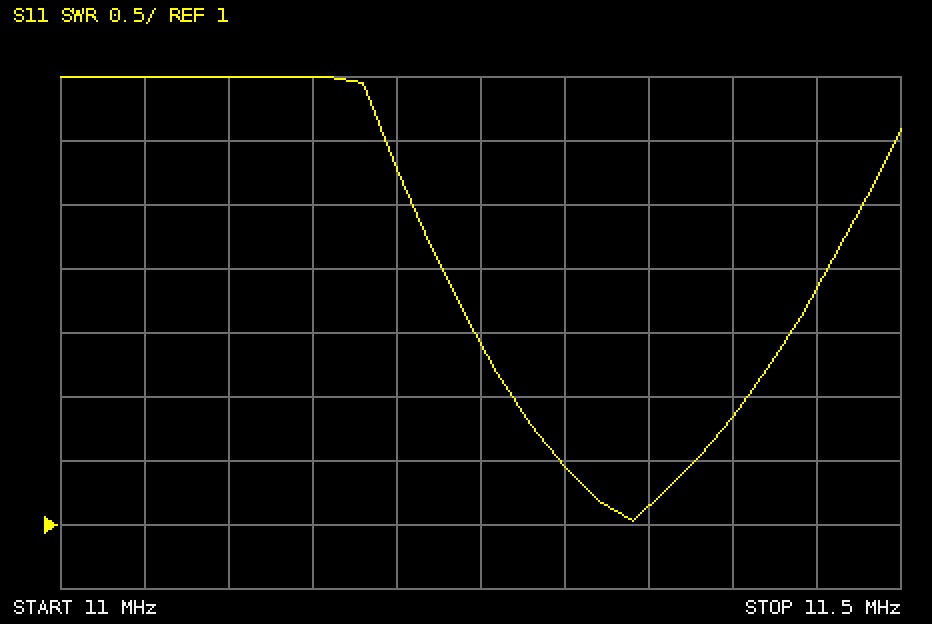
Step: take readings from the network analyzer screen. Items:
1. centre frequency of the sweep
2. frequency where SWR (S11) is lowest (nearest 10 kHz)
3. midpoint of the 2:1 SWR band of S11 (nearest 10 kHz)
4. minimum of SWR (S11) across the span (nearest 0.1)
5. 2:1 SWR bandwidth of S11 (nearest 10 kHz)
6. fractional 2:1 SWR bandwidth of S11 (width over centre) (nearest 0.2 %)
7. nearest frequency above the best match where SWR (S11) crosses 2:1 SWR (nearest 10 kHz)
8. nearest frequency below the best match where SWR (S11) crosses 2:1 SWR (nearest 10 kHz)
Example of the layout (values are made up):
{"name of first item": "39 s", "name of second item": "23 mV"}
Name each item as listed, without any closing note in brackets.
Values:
{"centre frequency of the sweep": "11.25 MHz", "frequency where SWR (S11) is lowest": "11.34 MHz", "midpoint of the 2:1 SWR band of S11": "11.34 MHz", "minimum of SWR (S11) across the span": "1.0", "2:1 SWR bandwidth of S11": "140 kHz", "fractional 2:1 SWR bandwidth of S11 (width over centre)": "1.2 %", "nearest frequency above the best match where SWR (S11) crosses 2:1 SWR": "11.41 MHz", "nearest frequency below the best match where SWR (S11) crosses 2:1 SWR": "11.27 MHz"}
